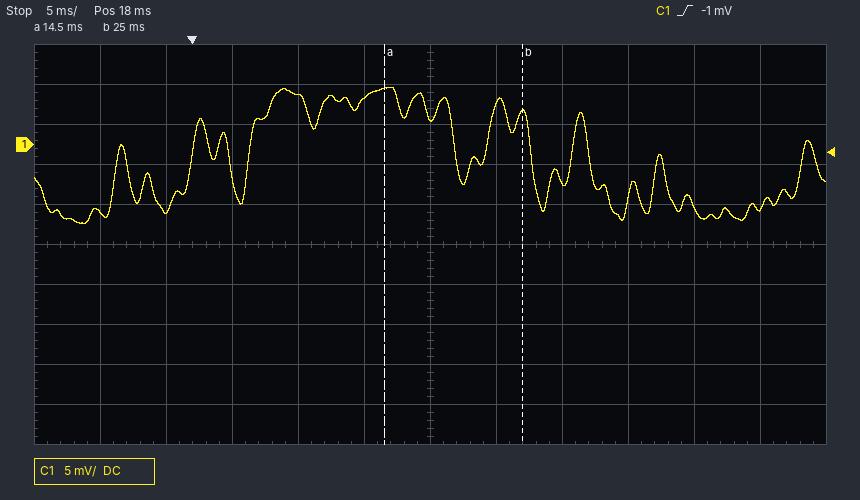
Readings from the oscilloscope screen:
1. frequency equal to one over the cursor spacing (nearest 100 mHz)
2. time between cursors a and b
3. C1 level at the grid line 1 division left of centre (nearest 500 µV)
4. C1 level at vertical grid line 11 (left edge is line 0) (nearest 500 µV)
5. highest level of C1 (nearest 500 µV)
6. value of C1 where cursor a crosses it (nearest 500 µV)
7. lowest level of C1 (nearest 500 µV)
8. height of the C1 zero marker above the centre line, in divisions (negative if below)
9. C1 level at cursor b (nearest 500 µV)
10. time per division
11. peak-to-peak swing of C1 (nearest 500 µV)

95.2 Hz
10.5 ms
6.0 mV
-8.0 mV
7.0 mV
7.0 mV
-10.0 mV
+2.5 div
4.0 mV
5 ms
17.0 mV
